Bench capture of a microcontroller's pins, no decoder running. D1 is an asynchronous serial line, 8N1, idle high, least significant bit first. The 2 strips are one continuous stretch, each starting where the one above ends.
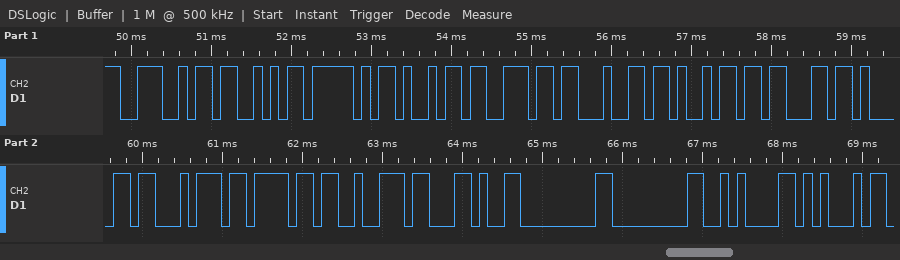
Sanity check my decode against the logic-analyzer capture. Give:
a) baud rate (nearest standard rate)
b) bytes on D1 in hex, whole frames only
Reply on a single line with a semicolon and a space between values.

9600 baud; 0x4E 0x53 0x5F 0x69 0x6E 0x64 0x69 0x63 0x61 0x74 0x6F 0x72 0x2C 0x00 0x00 0x0A 0x45
